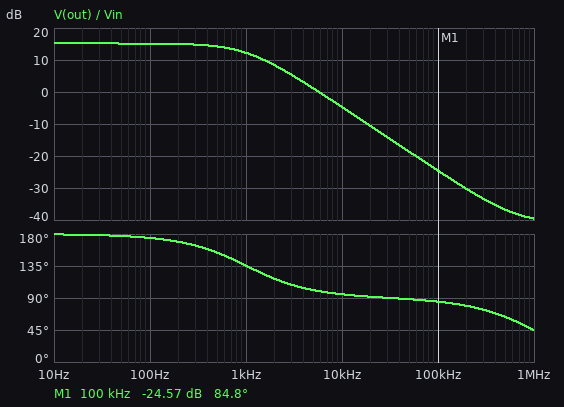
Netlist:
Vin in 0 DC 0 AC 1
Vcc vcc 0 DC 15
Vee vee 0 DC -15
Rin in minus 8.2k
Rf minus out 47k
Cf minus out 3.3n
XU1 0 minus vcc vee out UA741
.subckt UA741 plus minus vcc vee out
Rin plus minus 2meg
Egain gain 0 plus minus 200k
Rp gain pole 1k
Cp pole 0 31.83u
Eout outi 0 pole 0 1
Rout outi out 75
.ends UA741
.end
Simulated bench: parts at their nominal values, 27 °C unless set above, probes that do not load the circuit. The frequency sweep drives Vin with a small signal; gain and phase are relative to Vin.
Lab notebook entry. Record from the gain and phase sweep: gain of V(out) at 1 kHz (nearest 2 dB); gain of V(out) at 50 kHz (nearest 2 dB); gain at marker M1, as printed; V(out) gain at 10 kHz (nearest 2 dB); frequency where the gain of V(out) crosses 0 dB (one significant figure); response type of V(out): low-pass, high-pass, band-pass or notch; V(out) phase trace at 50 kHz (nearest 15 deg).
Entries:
12 dB
-18 dB
-24.57 dB
-4 dB
6 kHz
low-pass
90 deg
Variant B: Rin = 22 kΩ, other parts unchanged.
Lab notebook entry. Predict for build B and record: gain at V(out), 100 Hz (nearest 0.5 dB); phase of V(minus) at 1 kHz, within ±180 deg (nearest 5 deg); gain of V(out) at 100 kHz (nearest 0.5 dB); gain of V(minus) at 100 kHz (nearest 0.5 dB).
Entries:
6.5 dB
45 deg
-33.0 dB
-53.0 dB
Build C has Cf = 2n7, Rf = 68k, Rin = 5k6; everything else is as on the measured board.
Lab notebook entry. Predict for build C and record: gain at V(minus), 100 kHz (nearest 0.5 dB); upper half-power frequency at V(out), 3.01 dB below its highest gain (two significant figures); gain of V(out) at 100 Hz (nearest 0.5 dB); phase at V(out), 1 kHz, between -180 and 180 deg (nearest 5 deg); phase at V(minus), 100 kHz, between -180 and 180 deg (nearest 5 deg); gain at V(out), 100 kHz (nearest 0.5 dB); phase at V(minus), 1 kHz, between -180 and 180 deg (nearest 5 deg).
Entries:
-39.5 dB
860 Hz
21.5 dB
130 deg
0 deg
-19.5 dB
40 deg
